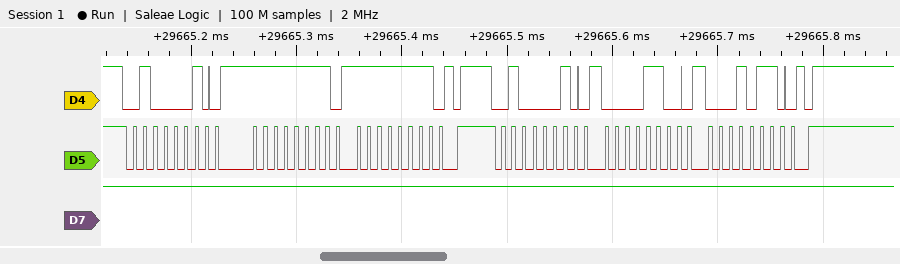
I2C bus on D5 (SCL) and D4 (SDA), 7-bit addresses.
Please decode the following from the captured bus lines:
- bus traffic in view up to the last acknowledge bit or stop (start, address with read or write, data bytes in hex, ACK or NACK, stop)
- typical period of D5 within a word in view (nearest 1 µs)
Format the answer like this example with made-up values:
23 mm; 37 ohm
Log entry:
start, address 21 write ACK, FF ACK, FF ACK, stop, start, address 21 write ACK, 0C ACK, 16 ACK, stop; 10 µs
